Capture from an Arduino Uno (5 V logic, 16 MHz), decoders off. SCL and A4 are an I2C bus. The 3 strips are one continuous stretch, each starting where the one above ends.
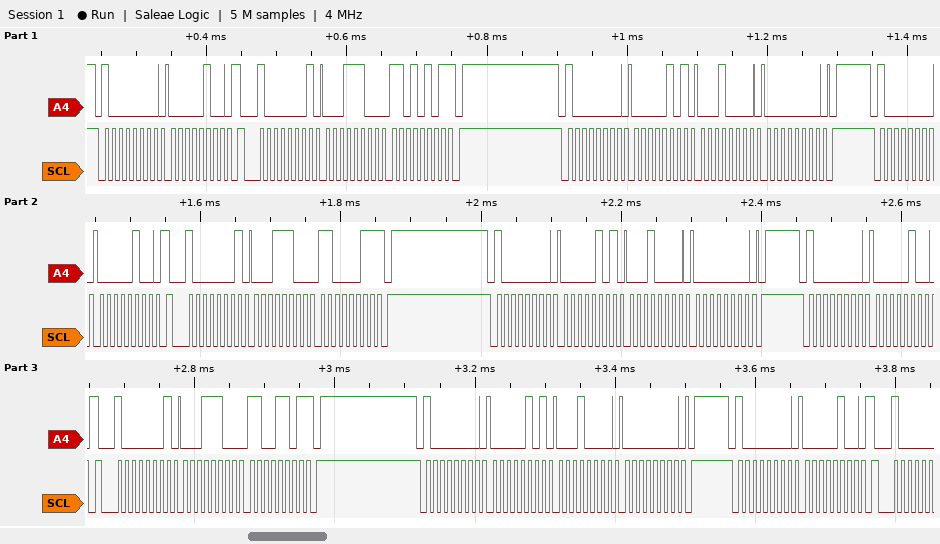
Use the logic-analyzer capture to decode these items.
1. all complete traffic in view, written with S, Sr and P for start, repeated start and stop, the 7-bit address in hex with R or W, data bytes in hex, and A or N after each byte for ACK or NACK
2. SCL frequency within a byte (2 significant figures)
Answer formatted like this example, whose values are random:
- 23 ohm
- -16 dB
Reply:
- S 40W A 04 A Sr 40R A 1C A D5 N P S 40W A 05 A 10 A 00 A P S 40W A 04 A Sr 40R A 1C A C3 N P S 40W A 05 A 10 A 00 A P S 40W A 04 A Sr 40R A 1C A CD N P S 40W A 05 A 10 A 00 A P S 40W A 04 A
- 100 kHz
